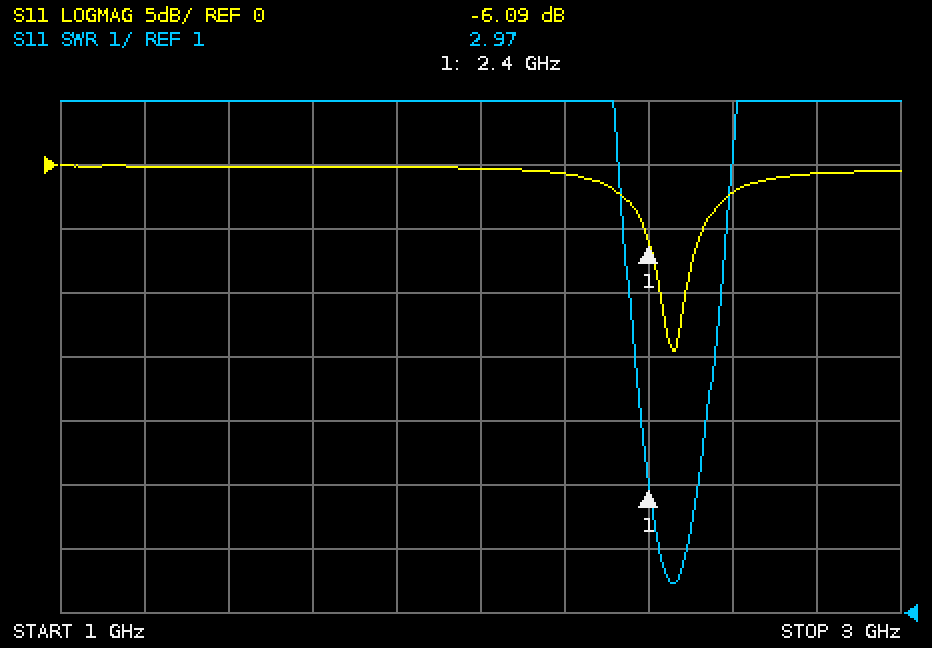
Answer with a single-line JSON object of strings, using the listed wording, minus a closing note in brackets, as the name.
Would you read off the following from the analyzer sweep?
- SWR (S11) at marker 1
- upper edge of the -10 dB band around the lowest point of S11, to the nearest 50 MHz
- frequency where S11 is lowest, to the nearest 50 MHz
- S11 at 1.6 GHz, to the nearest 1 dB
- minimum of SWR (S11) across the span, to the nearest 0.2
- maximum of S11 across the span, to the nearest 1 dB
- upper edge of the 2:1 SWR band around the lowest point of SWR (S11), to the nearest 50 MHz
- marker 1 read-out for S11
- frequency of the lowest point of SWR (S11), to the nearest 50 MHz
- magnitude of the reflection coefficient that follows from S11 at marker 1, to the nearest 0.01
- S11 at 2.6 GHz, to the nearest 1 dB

{"SWR (S11) at marker 1": "2.97", "upper edge of the -10 dB band around the lowest point of S11, to the nearest 50 MHz": "2.50 GHz", "frequency where S11 is lowest, to the nearest 50 MHz": "2.45 GHz", "S11 at 1.6 GHz, to the nearest 1 dB": "0 dB", "minimum of SWR (S11) across the span, to the nearest 0.2": "1.4", "maximum of S11 across the span, to the nearest 1 dB": "0 dB", "upper edge of the 2:1 SWR band around the lowest point of SWR (S11), to the nearest 50 MHz": "2.50 GHz", "marker 1 read-out for S11": "-6.09 dB", "frequency of the lowest point of SWR (S11), to the nearest 50 MHz": "2.45 GHz", "magnitude of the reflection coefficient that follows from S11 at marker 1, to the nearest 0.01": "0.50", "S11 at 2.6 GHz, to the nearest 1 dB": "-2 dB"}
